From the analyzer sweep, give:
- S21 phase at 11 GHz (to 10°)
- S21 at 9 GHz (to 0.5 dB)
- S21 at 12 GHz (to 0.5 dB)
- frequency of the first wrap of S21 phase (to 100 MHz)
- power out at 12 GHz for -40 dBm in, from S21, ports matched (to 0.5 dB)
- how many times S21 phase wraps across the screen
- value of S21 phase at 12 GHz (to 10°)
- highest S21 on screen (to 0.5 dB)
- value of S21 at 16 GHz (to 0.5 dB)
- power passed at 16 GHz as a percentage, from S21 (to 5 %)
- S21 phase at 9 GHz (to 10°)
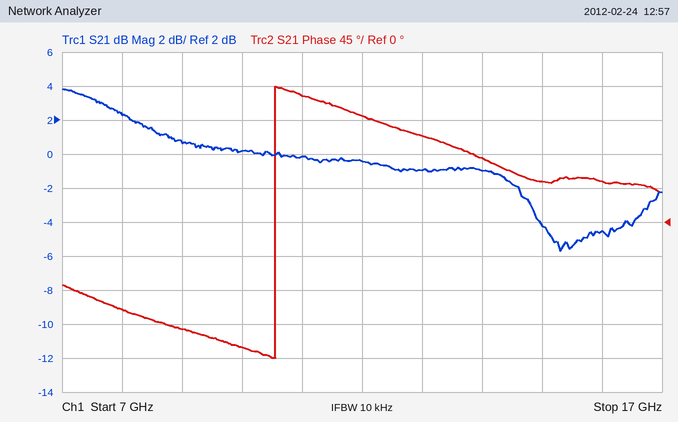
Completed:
170°
0.5 dB
-0.5 dB
10.6 GHz
-40.5 dBm
1
140°
4.0 dB
-4.5 dB
35 %
-140°
